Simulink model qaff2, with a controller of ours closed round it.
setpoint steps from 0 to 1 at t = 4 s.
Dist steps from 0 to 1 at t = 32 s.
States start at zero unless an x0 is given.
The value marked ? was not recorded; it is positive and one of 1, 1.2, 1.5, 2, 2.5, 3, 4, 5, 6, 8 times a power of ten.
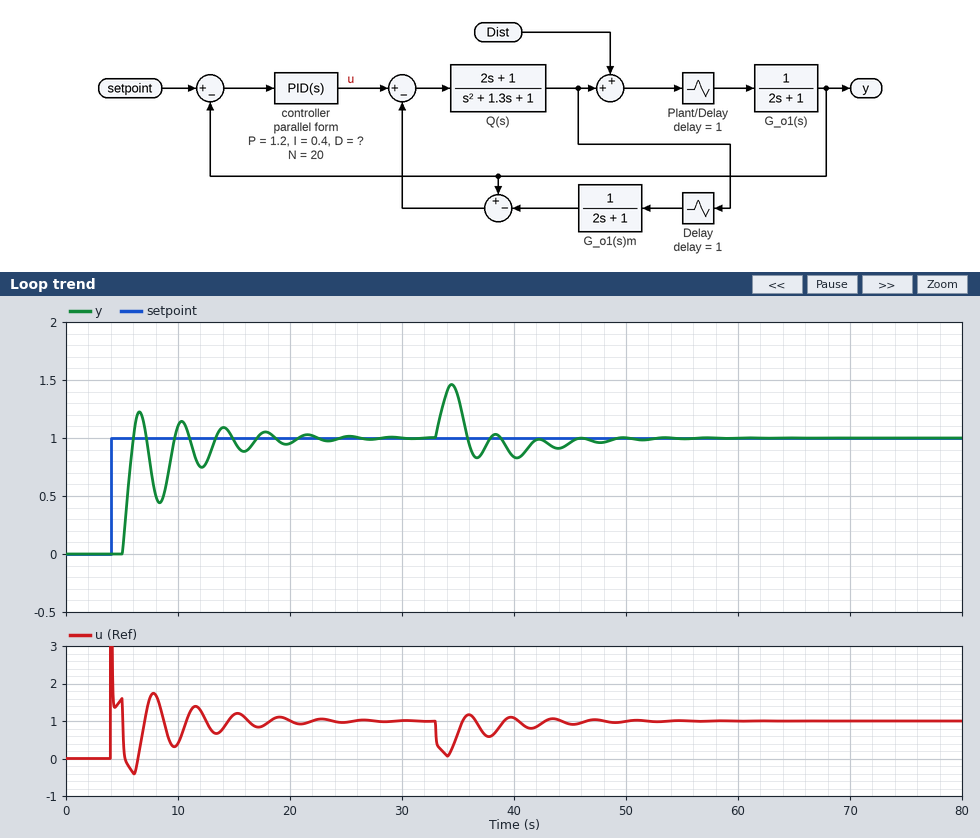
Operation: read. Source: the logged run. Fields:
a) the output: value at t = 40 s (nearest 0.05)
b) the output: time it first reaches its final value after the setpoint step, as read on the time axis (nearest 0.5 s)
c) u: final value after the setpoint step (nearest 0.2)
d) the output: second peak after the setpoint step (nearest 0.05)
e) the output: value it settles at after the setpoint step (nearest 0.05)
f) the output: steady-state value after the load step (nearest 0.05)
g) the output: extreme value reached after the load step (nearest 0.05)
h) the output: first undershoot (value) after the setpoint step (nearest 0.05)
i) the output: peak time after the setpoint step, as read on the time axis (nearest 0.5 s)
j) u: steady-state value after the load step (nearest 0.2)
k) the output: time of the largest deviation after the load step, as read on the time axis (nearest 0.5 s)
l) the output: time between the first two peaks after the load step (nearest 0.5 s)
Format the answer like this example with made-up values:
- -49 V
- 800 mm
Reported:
- 0.85
- 6.0 s
- 1.0
- 1.15
- 1.00
- 1.00
- 1.45
- 0.45
- 6.5 s
- 1.0
- 34.5 s
- 4.0 s
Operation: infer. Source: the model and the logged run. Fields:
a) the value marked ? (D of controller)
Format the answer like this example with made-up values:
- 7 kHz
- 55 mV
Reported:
- 1.2
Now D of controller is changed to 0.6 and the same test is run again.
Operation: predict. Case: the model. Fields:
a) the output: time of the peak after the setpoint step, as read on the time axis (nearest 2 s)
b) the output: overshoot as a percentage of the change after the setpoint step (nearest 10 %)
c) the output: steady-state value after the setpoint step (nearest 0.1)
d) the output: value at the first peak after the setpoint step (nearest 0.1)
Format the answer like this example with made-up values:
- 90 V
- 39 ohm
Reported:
- 8 s
- 20 %
- 1.0
- 1.2
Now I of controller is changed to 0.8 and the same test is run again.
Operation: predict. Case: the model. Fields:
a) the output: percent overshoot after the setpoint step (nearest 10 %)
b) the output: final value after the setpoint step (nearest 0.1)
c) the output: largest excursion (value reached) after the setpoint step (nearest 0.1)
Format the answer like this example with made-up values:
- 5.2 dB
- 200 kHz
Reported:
- 40 %
- 1.0
- 1.4
